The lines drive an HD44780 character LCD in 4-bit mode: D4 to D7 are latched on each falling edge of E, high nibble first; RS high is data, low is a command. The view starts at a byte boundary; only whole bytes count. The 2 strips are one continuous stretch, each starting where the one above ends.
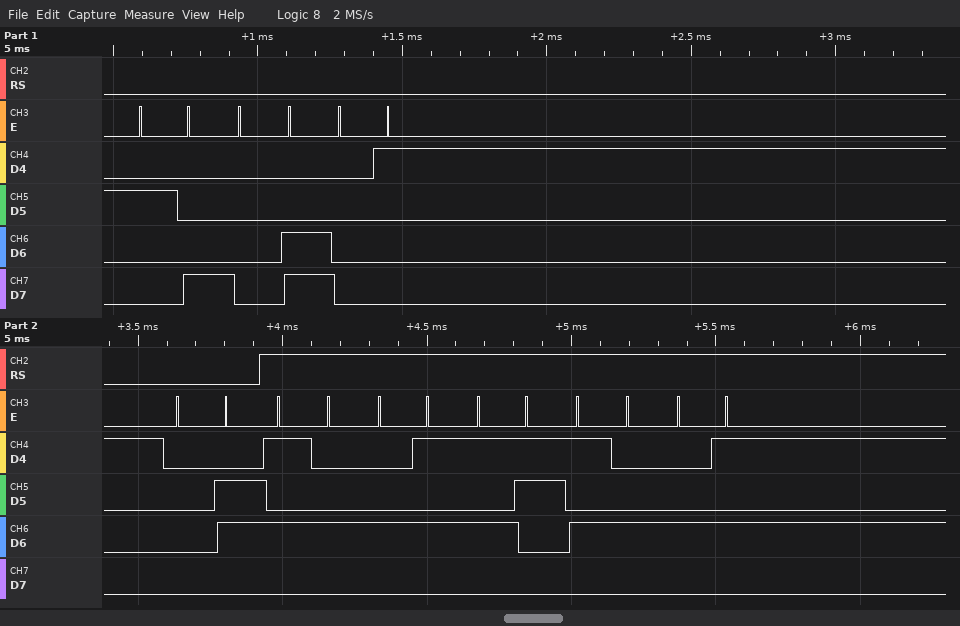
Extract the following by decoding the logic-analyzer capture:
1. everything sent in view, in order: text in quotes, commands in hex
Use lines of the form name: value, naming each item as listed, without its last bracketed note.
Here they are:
everything sent in view, in order: text in quotes, commands in hex: 0x28 0x0C 0x01 0x06 "TESTE"
